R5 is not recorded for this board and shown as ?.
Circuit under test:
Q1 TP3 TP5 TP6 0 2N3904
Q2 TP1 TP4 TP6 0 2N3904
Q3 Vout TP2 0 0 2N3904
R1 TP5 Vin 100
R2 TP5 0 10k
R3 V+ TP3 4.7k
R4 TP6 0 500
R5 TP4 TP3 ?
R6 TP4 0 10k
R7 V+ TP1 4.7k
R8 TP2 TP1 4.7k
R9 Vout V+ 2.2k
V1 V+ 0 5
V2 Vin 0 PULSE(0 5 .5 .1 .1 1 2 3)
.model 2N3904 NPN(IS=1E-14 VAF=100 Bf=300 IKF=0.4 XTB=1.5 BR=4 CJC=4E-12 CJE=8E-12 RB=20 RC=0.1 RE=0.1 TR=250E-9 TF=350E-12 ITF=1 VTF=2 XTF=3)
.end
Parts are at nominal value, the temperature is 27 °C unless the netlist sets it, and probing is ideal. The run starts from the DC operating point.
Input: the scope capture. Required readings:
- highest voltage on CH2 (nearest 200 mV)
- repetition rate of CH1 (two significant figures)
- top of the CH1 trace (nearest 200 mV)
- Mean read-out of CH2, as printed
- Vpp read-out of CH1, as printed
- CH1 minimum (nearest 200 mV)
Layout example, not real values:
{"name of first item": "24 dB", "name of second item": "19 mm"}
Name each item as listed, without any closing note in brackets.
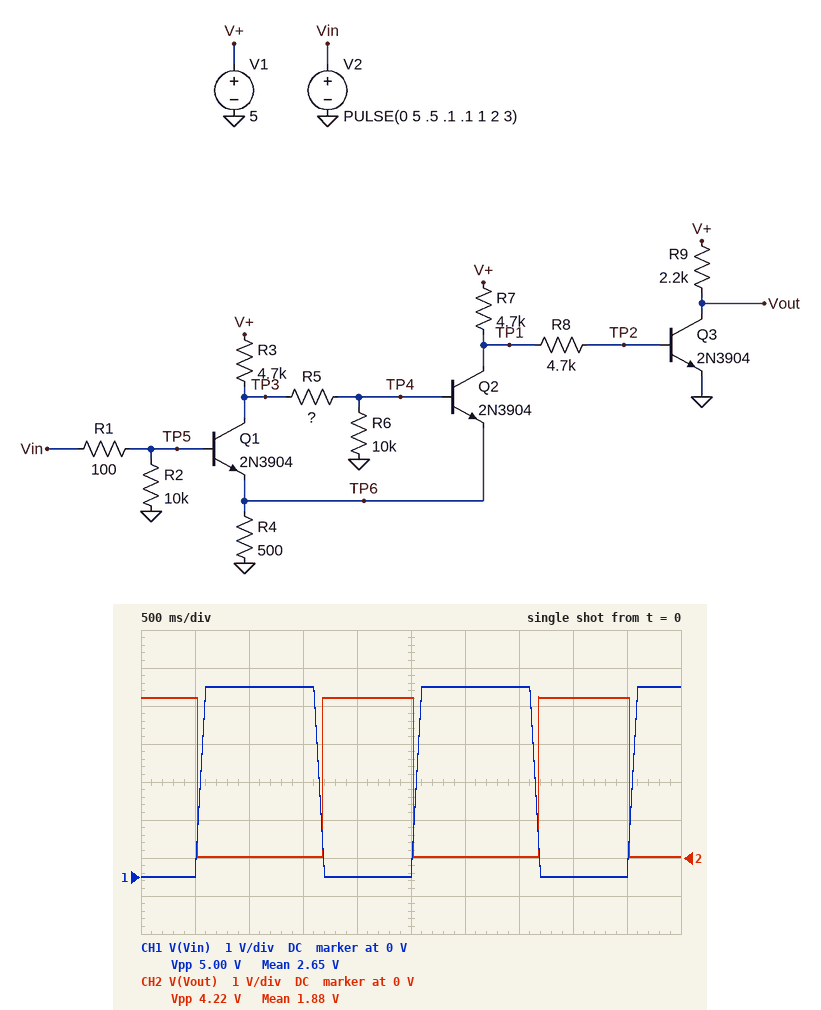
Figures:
{"highest voltage on CH2": "4.2 V", "repetition rate of CH1": "500 mHz", "top of the CH1 trace": "5.0 V", "Mean read-out of CH2, as printed": "1.88 V", "Vpp read-out of CH1, as printed": "5.00 V", "CH1 minimum": "0 V"}
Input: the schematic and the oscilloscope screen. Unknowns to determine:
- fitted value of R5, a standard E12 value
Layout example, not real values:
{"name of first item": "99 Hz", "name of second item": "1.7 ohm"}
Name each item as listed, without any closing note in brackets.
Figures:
{"fitted value of R5, a standard E12 value": "3.9 kΩ"}
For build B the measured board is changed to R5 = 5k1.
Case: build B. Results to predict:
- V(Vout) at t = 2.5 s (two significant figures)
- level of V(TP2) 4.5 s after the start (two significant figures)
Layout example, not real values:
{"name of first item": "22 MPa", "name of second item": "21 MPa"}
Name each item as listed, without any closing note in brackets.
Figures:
{"V(Vout) at t = 2.5 s": "4.6 V", "level of V(TP2) 4.5 s after the start": "610 mV"}
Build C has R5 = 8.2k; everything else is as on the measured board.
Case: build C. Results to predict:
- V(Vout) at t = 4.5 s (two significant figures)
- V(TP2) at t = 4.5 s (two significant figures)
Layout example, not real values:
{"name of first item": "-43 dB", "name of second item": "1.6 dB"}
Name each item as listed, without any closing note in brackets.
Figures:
{"V(Vout) at t = 4.5 s": "4.9 V", "V(TP2) at t = 4.5 s": "580 mV"}
